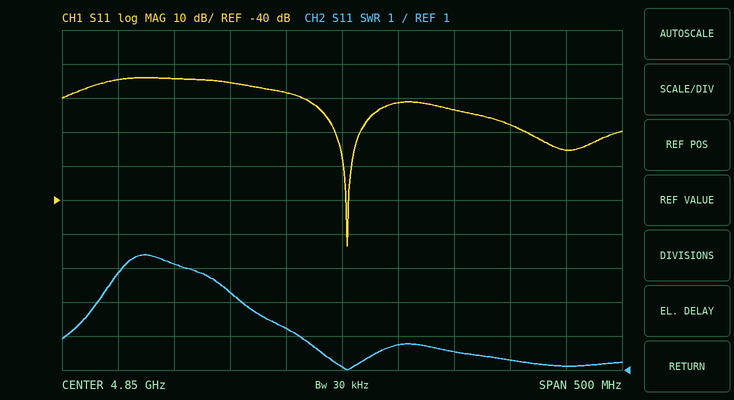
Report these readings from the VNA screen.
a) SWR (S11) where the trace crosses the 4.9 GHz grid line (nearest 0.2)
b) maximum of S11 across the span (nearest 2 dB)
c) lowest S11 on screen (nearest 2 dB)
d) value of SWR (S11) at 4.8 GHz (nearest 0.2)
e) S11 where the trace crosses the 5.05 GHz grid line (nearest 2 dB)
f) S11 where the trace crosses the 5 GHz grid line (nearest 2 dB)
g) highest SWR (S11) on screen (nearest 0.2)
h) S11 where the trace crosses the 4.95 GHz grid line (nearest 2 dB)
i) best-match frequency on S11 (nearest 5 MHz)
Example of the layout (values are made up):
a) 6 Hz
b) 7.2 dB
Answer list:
a) 1.8
b) -4 dB
c) -54 dB
d) 2.2
e) -26 dB
f) -18 dB
g) 4.4
h) -14 dB
i) 4.855 GHz
